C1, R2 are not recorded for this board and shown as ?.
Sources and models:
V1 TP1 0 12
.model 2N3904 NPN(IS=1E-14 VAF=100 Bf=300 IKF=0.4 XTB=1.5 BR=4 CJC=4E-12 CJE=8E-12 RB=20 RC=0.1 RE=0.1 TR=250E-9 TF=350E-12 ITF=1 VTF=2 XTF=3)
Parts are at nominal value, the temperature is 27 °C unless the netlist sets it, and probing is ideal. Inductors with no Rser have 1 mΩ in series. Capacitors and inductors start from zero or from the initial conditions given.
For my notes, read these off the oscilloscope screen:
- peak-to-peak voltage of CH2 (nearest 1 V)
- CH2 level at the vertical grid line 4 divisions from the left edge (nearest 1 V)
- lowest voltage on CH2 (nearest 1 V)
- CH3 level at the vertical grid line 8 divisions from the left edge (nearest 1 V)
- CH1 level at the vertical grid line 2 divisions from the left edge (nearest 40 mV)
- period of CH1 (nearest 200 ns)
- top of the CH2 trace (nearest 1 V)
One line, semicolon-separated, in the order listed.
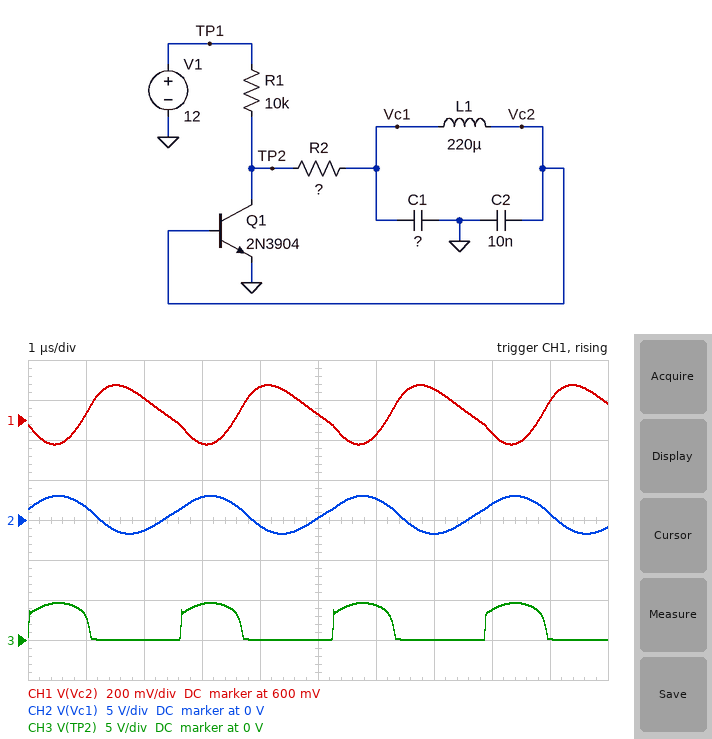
5 V; -1 V; -2 V; 4 V; 720 mV; 2.6 µs; 3 V
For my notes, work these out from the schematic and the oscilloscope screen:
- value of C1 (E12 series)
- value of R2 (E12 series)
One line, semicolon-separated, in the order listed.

820 pF; 2.2 kΩ
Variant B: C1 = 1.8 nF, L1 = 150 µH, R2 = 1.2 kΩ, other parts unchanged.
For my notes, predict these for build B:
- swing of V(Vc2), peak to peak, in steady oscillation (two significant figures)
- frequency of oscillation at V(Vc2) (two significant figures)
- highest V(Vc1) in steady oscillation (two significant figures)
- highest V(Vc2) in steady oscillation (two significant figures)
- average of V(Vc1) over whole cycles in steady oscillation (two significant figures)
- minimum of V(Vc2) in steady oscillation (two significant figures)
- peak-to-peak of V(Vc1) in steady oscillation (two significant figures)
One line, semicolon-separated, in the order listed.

450 mV; 320 kHz; 2.2 V; 800 mV; 590 mV; 350 mV; 3.2 V
